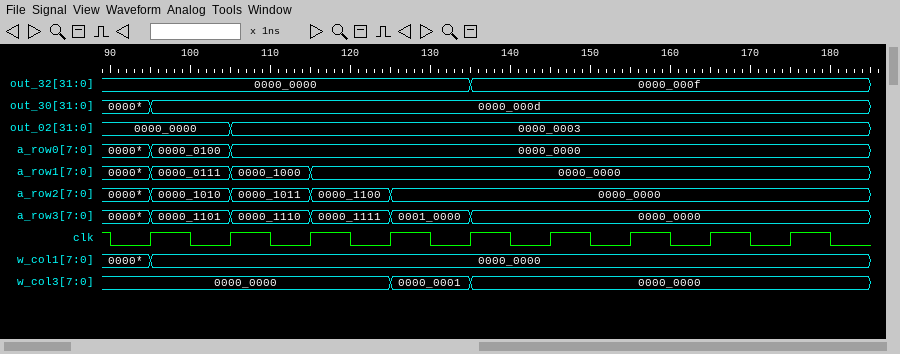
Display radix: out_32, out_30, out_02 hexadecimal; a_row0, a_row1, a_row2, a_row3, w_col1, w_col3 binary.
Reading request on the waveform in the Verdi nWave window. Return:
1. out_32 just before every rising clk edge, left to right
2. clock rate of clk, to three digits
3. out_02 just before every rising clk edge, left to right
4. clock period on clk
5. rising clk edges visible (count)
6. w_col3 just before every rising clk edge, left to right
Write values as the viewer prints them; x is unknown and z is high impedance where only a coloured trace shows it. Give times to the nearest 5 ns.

0000_0000, 0000_0000, 0000_0000, 0000_0000, 0000_0000, 0000_000f, 0000_000f, 0000_000f, 0000_000f
100 MHz
0000_0000, 0000_0000, 0000_0003, 0000_0003, 0000_0003, 0000_0003, 0000_0003, 0000_0003, 0000_0003
10 ns
9
0000_0000, 0000_0000, 0000_0000, 0000_0000, 0000_0001, 0000_0000, 0000_0000, 0000_0000, 0000_0000
